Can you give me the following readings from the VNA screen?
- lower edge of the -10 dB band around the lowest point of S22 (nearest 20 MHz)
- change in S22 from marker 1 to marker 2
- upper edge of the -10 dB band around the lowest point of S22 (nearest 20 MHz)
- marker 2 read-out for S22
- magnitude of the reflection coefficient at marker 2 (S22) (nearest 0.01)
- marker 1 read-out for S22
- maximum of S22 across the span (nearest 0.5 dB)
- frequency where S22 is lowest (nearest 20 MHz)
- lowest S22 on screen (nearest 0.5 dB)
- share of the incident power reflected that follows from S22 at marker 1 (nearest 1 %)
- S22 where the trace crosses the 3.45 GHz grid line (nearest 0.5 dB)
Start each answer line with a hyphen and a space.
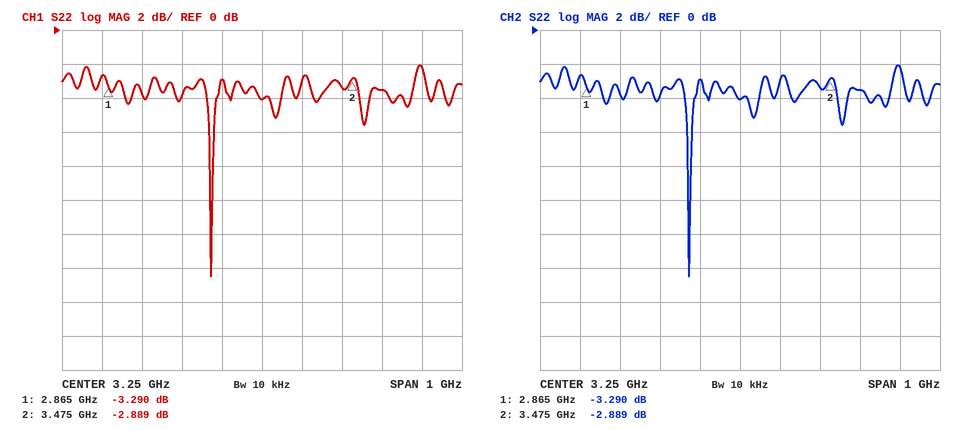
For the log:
- 3.12 GHz
- 0.401 dB
- 3.12 GHz
- -2.889 dB
- 0.72
- -3.290 dB
- -2.0 dB
- 3.12 GHz
- -14.5 dB
- 47 %
- -3.5 dB
